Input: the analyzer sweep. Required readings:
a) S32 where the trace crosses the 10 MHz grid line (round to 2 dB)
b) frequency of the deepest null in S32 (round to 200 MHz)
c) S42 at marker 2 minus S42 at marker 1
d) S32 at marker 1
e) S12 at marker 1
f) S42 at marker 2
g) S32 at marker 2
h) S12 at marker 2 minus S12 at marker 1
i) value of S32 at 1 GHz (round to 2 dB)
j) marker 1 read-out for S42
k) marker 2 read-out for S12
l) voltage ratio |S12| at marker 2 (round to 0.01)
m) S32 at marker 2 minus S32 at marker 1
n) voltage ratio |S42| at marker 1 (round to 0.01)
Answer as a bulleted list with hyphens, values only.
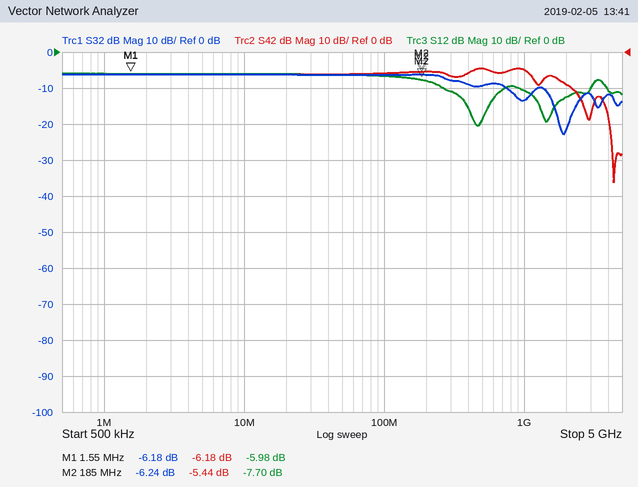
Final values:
- -6 dB
- 2.0 GHz
- 0.74 dB
- -6.18 dB
- -5.98 dB
- -5.44 dB
- -6.24 dB
- -1.72 dB
- -14 dB
- -6.18 dB
- -7.70 dB
- 0.41
- -0.06 dB
- 0.49
